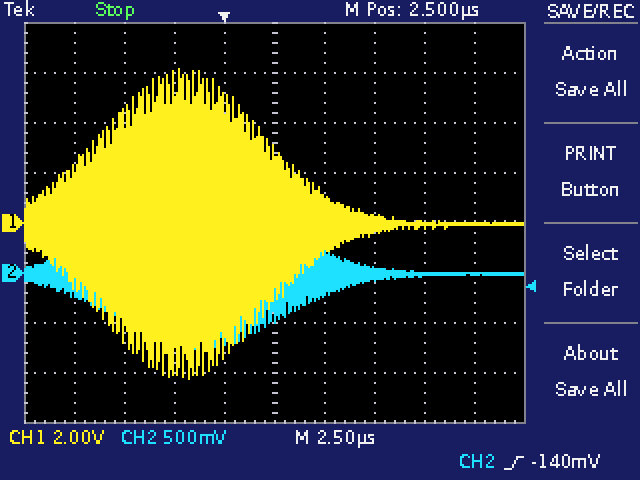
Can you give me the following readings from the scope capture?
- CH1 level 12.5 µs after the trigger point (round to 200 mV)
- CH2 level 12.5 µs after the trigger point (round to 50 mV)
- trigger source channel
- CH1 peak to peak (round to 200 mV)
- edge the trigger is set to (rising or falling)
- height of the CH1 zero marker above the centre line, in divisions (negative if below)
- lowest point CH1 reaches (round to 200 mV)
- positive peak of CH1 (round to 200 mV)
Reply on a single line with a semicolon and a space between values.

0.0 V; 0 mV; CH2; 12.4 V; rising; 0.0 div; -6.2 V; 6.2 V
